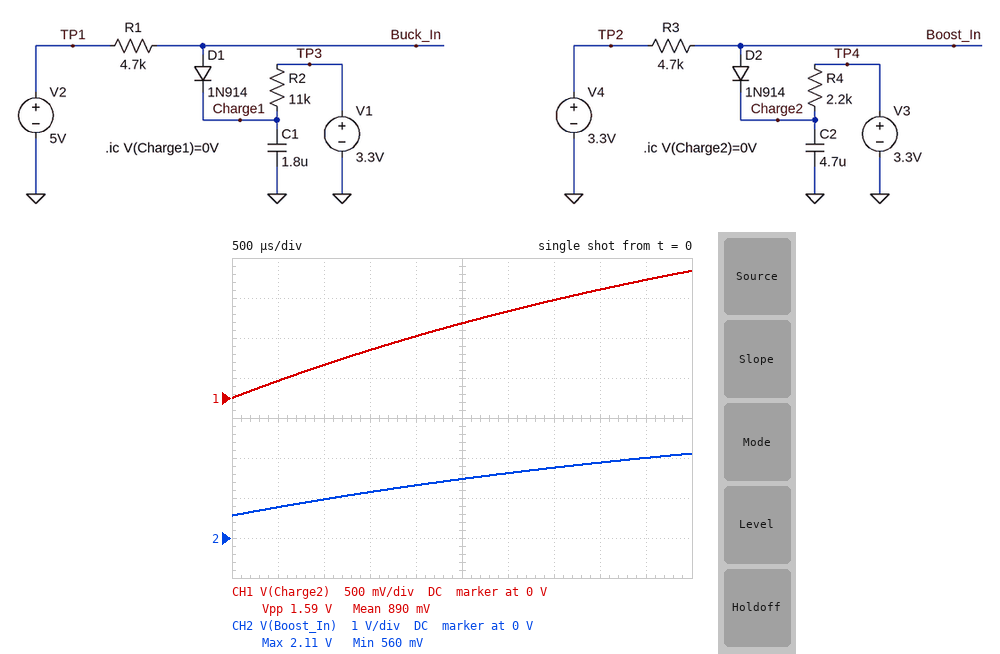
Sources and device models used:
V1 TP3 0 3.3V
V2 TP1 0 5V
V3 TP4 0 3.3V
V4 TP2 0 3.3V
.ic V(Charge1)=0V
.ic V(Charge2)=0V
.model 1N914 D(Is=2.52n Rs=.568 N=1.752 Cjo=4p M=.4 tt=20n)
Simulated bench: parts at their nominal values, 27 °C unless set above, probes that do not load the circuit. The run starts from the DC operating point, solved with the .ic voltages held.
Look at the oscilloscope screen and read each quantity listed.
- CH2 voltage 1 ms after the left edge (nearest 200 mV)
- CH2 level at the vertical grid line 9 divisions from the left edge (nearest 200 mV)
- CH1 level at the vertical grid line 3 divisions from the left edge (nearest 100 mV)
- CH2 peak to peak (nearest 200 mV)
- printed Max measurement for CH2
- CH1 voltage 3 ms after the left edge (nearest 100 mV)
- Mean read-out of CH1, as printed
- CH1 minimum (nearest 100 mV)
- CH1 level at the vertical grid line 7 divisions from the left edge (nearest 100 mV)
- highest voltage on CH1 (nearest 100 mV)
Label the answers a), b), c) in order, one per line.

a) 1.0 V
b) 2.0 V
c) 600 mV
d) 1.6 V
e) 2.11 V
f) 1.1 V
g) 890 mV
h) 0 V
i) 1.2 V
j) 1.6 V
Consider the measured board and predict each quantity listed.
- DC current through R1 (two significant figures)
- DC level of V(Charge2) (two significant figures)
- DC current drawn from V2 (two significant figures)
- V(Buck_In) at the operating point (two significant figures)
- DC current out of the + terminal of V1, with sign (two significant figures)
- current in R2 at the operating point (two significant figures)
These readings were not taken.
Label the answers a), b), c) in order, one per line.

a) 78 µA
b) 3.3 V
c) 78 µA
d) 4.6 V
e) -78 µA
f) 78 µA
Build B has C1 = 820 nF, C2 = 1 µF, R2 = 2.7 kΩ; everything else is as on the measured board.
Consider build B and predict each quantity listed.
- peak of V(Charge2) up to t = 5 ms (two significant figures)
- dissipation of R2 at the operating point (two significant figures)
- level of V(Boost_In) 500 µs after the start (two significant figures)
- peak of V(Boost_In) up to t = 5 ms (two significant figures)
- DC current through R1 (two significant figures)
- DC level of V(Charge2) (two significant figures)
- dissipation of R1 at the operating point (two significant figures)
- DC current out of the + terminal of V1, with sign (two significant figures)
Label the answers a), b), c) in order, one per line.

a) 3.1 V
b) 71 µW
c) 1.4 V
d) 3.3 V
e) 160 µA
f) 3.3 V
g) 120 µW
h) -160 µA
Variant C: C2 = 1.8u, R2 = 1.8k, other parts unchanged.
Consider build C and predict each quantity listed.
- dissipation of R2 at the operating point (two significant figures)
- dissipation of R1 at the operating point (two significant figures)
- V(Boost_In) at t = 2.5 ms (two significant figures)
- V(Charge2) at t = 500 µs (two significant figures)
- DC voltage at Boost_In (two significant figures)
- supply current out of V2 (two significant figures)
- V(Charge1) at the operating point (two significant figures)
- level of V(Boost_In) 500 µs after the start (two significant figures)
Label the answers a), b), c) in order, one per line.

a) 61 µW
b) 160 µW
c) 2.4 V
d) 530 mV
e) 3.3 V
f) 180 µA
g) 3.6 V
h) 1.1 V
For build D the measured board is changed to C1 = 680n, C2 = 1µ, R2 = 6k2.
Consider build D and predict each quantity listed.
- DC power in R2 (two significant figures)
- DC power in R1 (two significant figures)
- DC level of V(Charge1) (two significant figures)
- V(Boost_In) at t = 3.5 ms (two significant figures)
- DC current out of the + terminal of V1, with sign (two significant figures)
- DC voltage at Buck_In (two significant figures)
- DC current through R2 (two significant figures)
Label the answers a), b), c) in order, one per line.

a) 77 µW
b) 58 µW
c) 4.0 V
d) 3.2 V
e) -110 µA
f) 4.5 V
g) 110 µA
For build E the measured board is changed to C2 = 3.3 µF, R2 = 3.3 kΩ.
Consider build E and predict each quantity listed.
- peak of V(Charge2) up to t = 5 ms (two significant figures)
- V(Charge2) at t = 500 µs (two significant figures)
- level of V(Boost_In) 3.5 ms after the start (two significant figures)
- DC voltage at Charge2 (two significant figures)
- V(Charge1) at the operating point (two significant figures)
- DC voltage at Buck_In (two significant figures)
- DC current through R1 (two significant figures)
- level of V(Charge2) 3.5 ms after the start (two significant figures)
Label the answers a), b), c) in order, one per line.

a) 2.0 V
b) 300 mV
c) 2.1 V
d) 3.3 V
e) 3.8 V
f) 4.3 V
g) 150 µA
h) 1.6 V
